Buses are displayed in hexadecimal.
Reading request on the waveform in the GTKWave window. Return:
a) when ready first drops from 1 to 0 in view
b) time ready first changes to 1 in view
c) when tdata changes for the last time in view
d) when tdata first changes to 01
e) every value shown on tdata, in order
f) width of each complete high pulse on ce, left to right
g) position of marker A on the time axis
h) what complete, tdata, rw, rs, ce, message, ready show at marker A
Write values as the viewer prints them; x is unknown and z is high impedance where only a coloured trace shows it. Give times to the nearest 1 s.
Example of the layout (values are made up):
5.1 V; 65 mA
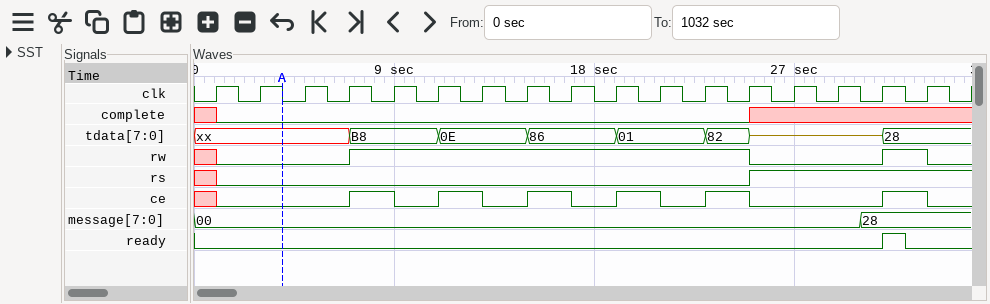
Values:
32 s; 31 s; 31 s; 19 s; xx, B8, 0E, 86, 01, 82, z, 28; 2 s, 2 s, 2 s, 2 s, 2 s, 2 s; 4 s; complete=0, tdata=xx, rw=0, rs=0, ce=0, message=00, ready=0
